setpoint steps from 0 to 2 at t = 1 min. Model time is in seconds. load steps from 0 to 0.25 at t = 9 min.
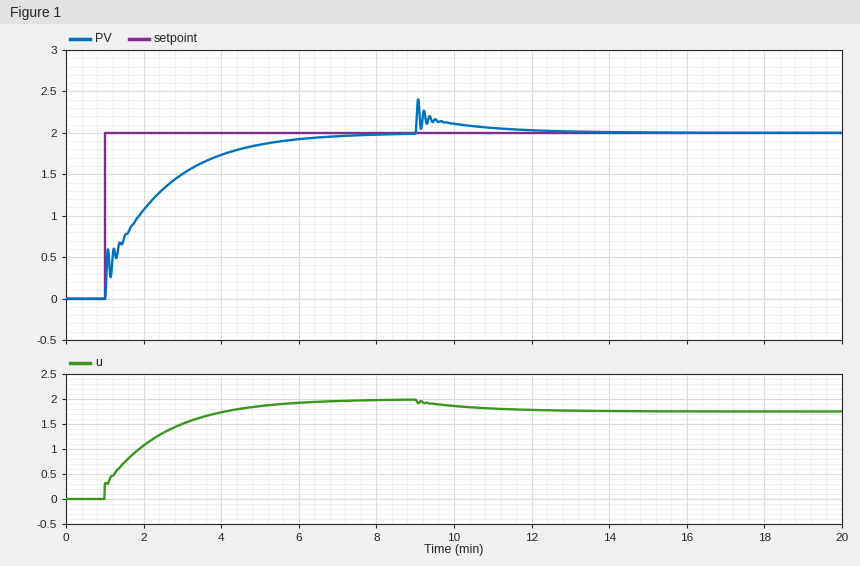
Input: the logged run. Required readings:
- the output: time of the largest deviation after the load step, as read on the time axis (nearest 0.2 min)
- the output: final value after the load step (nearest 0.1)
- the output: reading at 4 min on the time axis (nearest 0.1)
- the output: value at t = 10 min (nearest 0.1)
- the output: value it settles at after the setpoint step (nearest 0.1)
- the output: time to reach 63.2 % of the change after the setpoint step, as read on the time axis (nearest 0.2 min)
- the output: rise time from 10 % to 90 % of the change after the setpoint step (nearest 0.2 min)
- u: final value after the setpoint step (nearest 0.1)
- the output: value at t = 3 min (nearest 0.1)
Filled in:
9.0 min
2.0
1.7
2.1
2.0
2.4 min
3.4 min
2.0
1.5
